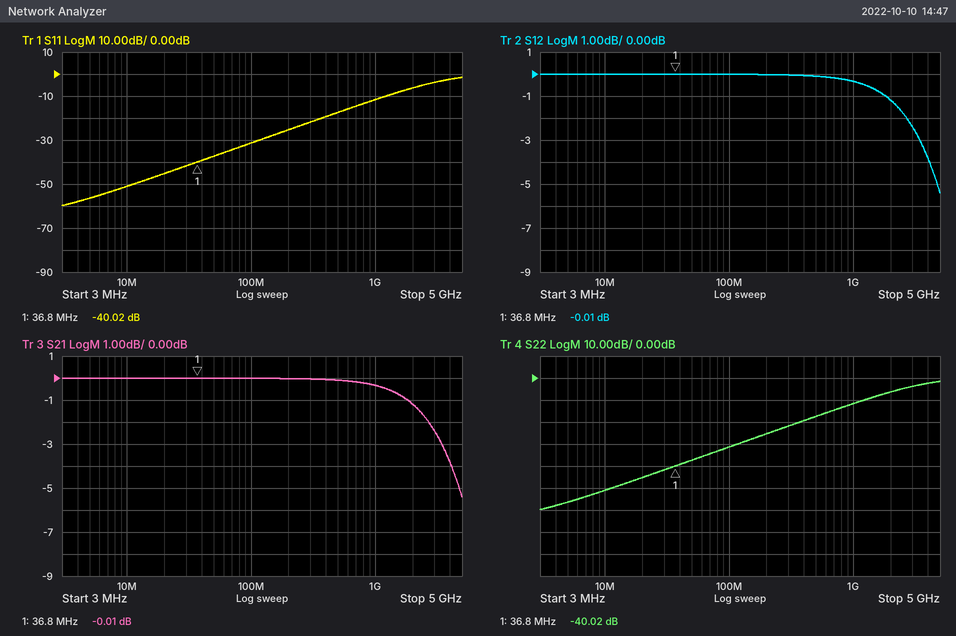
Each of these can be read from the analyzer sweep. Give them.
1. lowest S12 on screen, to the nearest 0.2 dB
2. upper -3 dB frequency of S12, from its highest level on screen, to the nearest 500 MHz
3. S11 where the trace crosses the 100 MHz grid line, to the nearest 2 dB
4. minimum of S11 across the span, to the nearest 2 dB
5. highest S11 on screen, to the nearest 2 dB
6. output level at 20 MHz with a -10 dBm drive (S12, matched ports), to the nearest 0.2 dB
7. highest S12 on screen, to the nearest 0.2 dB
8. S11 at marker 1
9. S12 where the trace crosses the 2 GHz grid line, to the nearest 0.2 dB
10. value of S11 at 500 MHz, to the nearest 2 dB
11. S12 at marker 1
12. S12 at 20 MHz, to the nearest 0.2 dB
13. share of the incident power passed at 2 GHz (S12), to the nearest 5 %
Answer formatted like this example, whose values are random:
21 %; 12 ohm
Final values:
-5.4 dB; 3.5 GHz; -32 dB; -60 dB; -2 dB; -10.0 dBm; 0.0 dB; -40.02 dB; -1.2 dB; -18 dB; -0.01 dB; 0.0 dB; 75 %
